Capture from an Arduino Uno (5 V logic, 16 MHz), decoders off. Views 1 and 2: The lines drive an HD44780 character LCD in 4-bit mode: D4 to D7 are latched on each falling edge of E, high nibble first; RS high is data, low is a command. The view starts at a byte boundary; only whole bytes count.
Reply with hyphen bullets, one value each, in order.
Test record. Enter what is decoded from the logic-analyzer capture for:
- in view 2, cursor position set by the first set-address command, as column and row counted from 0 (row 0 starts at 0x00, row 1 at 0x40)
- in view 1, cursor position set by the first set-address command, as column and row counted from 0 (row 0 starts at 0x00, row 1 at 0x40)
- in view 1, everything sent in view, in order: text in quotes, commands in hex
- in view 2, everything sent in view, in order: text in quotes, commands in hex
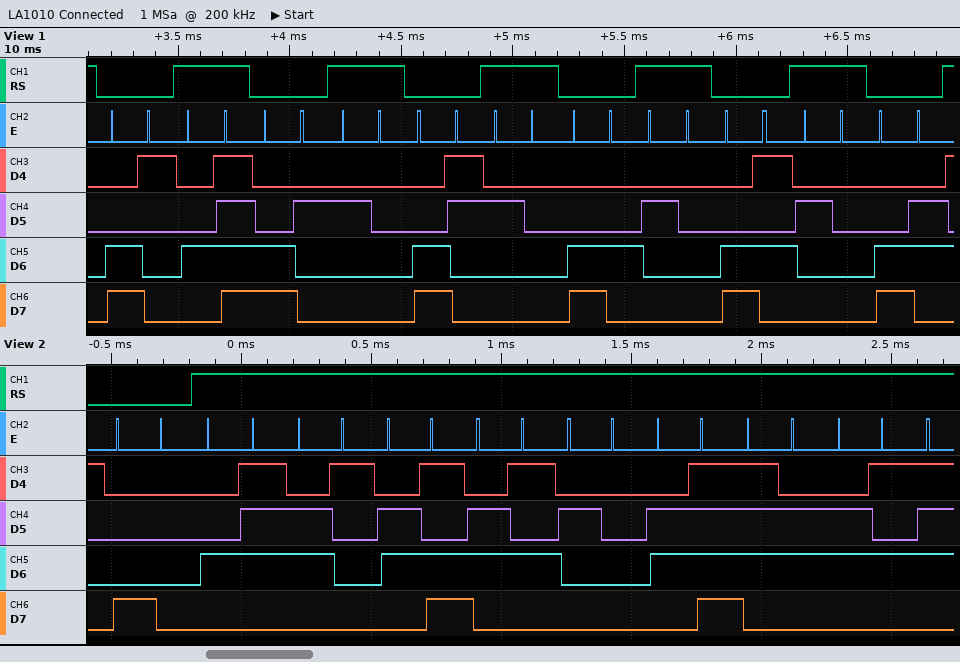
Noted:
- column 0, row 0
- column 1, row 1
- 0xC1 "O" 0xC2 " " 0xC3 " " 0xC4 " " 0xC5 " " 0xC6
- 0x80 "Game ove"
